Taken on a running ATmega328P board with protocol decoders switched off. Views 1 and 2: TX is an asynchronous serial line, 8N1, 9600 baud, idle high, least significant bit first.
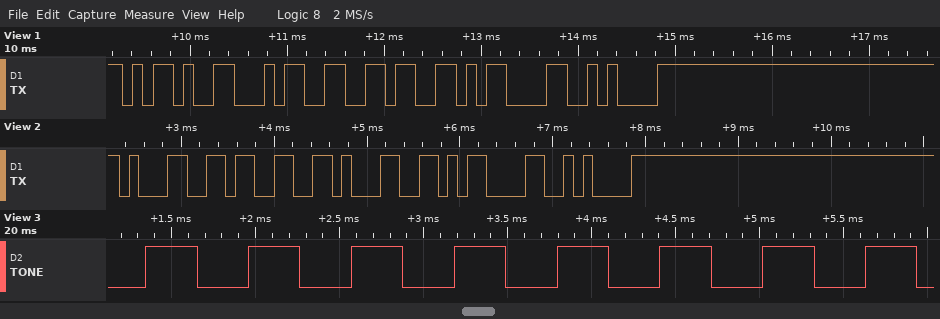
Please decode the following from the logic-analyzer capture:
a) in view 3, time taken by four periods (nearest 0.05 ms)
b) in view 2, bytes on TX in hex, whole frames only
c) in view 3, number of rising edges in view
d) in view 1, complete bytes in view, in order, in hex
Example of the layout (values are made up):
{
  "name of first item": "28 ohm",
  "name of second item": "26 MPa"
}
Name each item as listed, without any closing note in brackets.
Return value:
{
  "in view 3, time taken by four periods": "2.45 ms",
  "in view 2, bytes on TX in hex, whole frames only": "0x31 0x33 0x31 0x0D 0x0A",
  "in view 3, number of rising edges in view": "8",
  "in view 1, complete bytes in view, in order, in hex": "2D 34 36 0D 0A"
}
